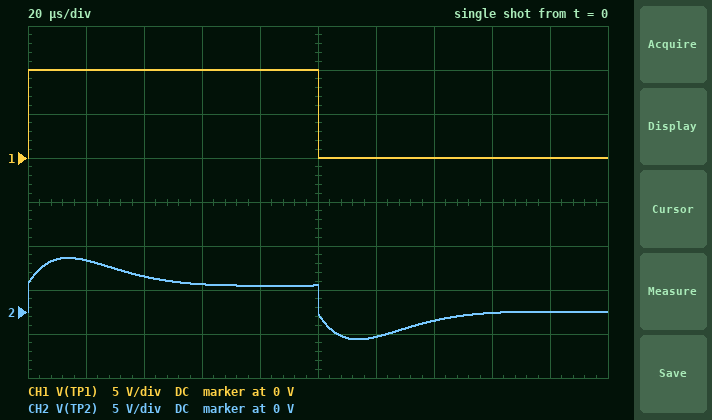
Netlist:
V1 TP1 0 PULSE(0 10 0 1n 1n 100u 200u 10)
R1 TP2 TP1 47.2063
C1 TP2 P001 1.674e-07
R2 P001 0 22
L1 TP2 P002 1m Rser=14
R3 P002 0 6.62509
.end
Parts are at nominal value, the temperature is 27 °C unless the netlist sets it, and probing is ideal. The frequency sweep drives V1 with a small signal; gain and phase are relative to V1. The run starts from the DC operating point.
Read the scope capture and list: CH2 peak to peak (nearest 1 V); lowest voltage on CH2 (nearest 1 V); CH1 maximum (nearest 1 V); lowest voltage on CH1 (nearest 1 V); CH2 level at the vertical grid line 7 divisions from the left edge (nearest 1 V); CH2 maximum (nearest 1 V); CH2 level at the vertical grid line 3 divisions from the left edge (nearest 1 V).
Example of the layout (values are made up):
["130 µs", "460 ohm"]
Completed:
["9 V", "-3 V", "10 V", "0 V", "-1 V", "6 V", "3 V"]
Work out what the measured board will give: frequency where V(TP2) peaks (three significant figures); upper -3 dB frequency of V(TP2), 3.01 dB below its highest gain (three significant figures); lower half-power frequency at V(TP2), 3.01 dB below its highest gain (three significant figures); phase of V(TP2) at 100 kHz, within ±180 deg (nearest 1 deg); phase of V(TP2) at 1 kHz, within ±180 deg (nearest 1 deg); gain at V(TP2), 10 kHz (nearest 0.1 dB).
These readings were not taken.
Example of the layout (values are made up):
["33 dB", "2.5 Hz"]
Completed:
["12.2 kHz", "29.2 kHz", "5.19 kHz", "-14 deg", "11 deg", "-2.6 dB"]
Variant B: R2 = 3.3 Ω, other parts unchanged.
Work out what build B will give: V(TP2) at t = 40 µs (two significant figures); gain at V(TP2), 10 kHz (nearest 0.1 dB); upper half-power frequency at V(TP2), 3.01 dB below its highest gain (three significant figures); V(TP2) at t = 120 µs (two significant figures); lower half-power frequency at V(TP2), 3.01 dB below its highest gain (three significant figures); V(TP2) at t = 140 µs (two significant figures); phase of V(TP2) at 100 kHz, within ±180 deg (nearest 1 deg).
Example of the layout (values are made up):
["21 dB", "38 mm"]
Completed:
["3.9 V", "-2.0 dB", "28.9 kHz", "-3.4 V", "6.12 kHz", "-900 mV", "-60 deg"]
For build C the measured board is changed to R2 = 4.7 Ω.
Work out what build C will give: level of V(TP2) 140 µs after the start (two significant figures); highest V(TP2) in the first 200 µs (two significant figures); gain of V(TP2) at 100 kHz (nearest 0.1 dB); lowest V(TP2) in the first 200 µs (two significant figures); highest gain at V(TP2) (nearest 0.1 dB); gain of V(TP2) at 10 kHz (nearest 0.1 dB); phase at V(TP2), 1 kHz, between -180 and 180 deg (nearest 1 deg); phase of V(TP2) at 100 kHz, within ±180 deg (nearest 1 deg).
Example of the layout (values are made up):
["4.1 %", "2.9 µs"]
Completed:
["-910 mV", "6.7 V", "-13.8 dB", "-3.7 V", "-1.4 dB", "-2.0 dB", "11 deg", "-53 deg"]
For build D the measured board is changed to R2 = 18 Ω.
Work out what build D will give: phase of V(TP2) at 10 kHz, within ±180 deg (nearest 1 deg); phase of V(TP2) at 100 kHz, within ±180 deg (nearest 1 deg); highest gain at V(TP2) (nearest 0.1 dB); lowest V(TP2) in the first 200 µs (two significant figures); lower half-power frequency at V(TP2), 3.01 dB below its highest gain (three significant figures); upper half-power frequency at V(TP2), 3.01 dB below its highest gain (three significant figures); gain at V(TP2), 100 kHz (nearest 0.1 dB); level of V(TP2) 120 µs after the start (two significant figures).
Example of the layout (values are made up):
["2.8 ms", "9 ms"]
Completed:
["9 deg", "-18 deg", "-2.2 dB", "-3.2 V", "5.34 kHz", "28.4 kHz", "-10.1 dB", "-2.9 V"]
